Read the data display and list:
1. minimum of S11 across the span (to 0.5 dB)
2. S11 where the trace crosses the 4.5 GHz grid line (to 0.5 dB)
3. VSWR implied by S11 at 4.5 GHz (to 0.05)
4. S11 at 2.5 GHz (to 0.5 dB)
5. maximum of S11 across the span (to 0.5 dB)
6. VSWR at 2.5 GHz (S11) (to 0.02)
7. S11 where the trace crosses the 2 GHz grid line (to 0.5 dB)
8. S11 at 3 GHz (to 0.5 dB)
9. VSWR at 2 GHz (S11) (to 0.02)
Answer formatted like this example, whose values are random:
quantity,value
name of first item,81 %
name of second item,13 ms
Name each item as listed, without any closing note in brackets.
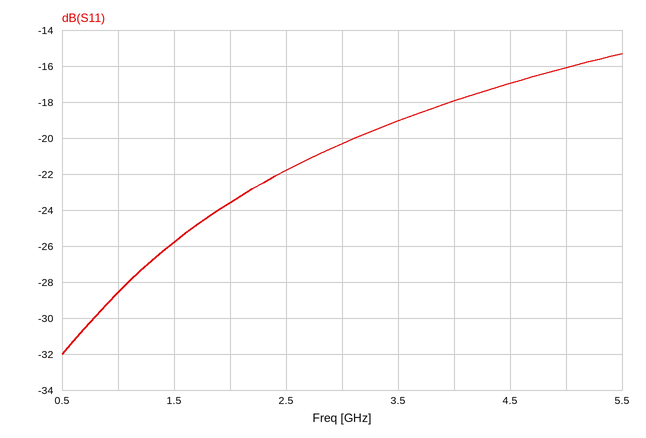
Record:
quantity,value
minimum of S11 across the span,-32.0 dB
S11 where the trace crosses the 4.5 GHz grid line,-17.0 dB
VSWR implied by S11 at 4.5 GHz,1.35
S11 at 2.5 GHz,-22.0 dB
maximum of S11 across the span,-15.5 dB
VSWR at 2.5 GHz (S11),1.18
S11 where the trace crosses the 2 GHz grid line,-23.5 dB
S11 at 3 GHz,-20.5 dB
VSWR at 2 GHz (S11),1.14
